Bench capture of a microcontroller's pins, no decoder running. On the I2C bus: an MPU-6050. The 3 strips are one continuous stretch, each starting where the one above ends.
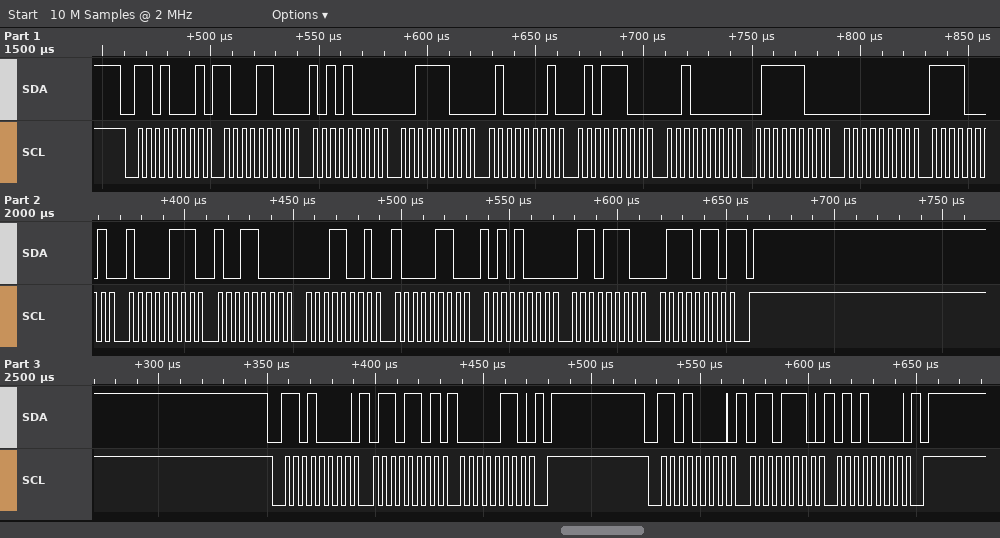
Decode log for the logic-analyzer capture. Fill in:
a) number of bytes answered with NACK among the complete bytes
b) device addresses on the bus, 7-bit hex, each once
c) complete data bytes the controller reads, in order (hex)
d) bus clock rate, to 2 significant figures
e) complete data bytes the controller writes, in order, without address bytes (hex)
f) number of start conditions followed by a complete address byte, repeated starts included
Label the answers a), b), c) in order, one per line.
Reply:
a) 1
b) 0x68
c) 8C A8 3C 41 5C 20 7C 00 F1 87 98 19 86 A8 6E 76
d) 250 kHz
e) 6D 06 6E 50
f) 3
